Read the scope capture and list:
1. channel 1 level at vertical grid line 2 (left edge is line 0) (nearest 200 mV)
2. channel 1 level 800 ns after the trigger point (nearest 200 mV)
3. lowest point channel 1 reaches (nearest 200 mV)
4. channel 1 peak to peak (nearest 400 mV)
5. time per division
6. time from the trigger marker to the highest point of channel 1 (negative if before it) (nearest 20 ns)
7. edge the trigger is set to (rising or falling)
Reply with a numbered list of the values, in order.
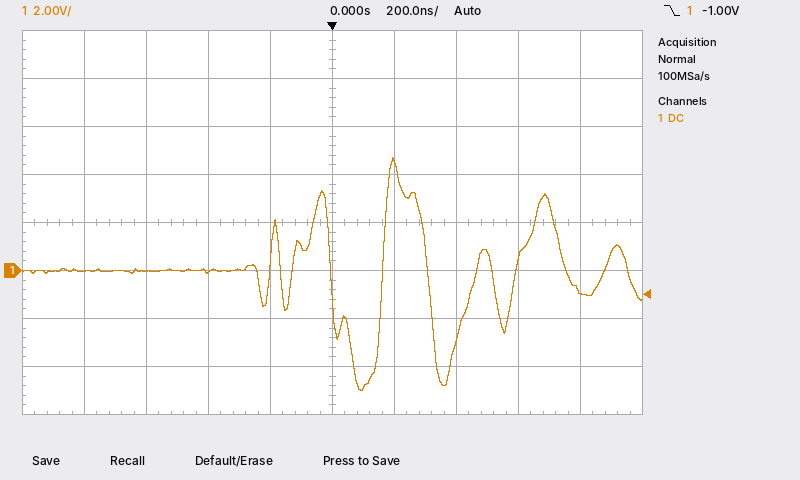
1. 0.0 V
2. -800 mV
3. -5.0 V
4. 9.6 V
5. 200 ns
6. +200 ns
7. falling
